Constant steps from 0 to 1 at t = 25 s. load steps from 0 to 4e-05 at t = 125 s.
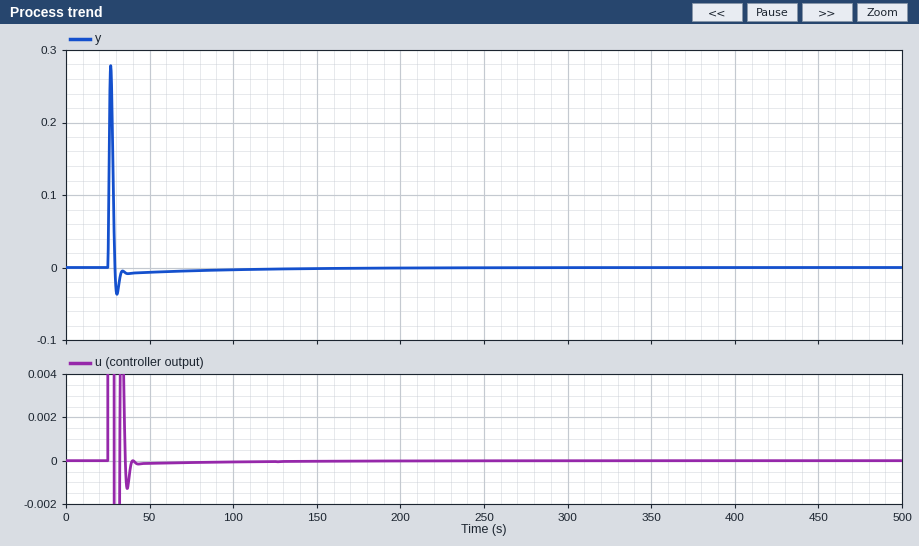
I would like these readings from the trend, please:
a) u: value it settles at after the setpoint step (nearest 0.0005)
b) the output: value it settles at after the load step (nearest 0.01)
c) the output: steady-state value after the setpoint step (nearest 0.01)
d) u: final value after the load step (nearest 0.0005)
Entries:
0.0000
0.00
0.00
0.0000
